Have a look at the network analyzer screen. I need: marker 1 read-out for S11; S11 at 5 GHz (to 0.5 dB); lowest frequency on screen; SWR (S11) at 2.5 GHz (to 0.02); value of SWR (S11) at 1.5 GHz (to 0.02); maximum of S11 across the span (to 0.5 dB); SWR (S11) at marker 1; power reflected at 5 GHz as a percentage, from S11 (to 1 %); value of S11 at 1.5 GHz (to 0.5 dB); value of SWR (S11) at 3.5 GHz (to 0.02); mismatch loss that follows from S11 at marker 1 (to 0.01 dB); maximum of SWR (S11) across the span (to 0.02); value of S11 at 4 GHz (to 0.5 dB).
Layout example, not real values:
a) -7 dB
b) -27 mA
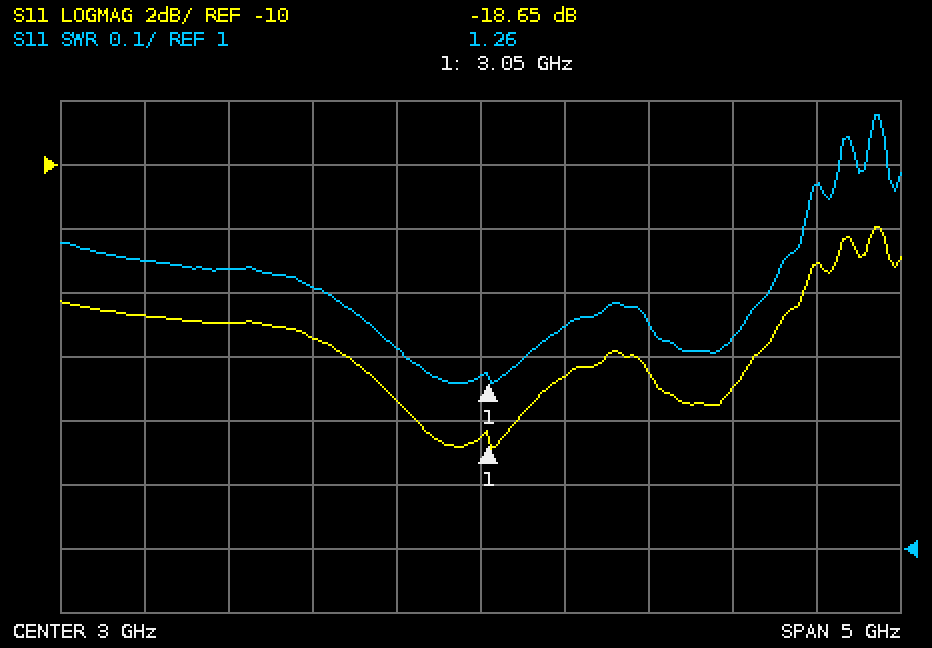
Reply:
a) -18.65 dB
b) -13.0 dB
c) 500 MHz
d) 1.32
e) 1.44
f) -12.0 dB
g) 1.26
h) 5 %
i) -15.0 dB
j) 1.34
k) 0.06 dB
l) 1.68
m) -16.5 dB
